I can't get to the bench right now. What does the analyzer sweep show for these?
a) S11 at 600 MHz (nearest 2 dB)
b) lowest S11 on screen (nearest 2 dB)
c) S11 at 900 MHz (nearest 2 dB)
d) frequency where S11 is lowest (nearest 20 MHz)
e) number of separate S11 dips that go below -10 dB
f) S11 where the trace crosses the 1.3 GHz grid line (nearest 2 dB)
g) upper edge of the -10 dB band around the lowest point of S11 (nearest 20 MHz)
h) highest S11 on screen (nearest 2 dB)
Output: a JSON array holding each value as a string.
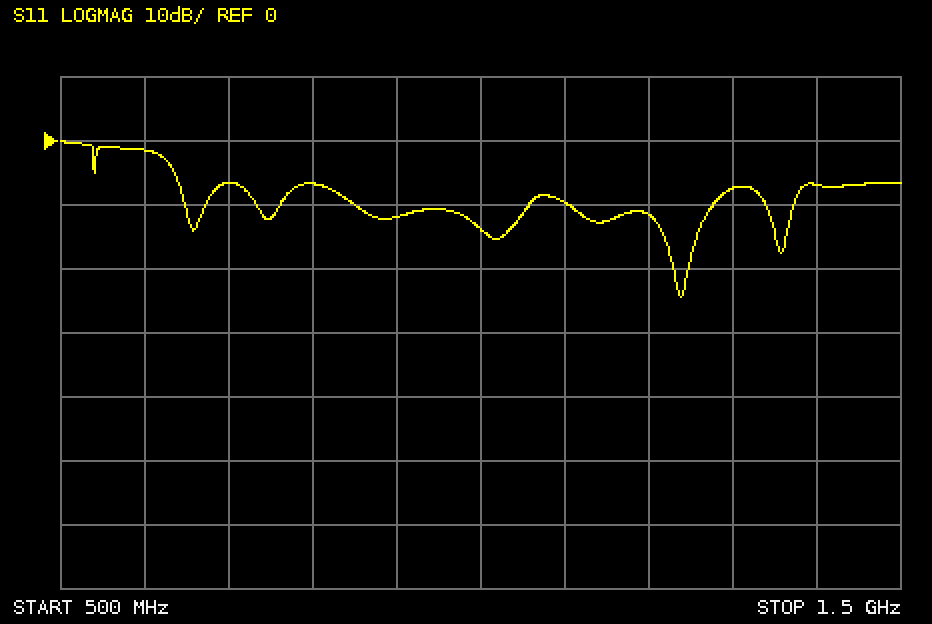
["-2 dB", "-24 dB", "-12 dB", "1.24 GHz", "5", "-8 dB", "1.28 GHz", "0 dB"]
